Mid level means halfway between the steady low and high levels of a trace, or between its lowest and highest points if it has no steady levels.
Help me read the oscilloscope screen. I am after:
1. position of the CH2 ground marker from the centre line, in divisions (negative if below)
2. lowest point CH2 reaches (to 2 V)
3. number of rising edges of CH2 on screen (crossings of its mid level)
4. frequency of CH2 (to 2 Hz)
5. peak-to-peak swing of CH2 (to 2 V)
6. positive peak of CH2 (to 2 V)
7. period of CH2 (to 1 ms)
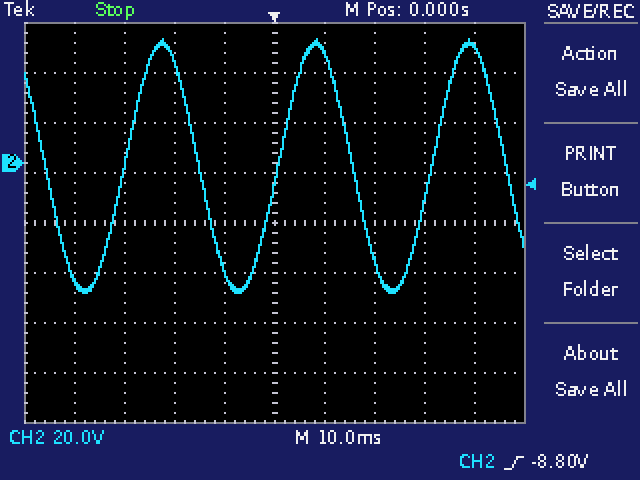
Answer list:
+1.2 div
-52 V
3
32 Hz
102 V
50 V
31 ms
